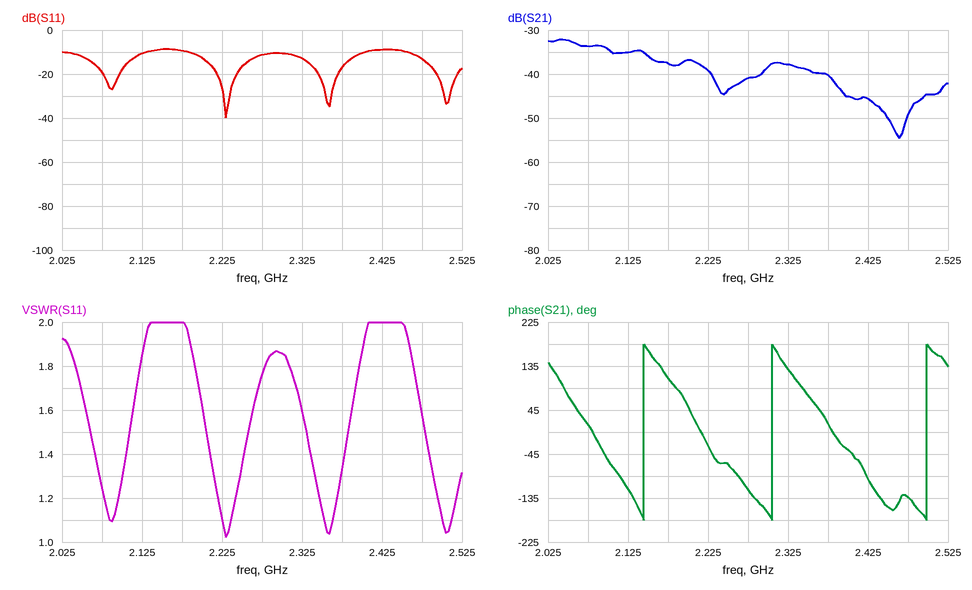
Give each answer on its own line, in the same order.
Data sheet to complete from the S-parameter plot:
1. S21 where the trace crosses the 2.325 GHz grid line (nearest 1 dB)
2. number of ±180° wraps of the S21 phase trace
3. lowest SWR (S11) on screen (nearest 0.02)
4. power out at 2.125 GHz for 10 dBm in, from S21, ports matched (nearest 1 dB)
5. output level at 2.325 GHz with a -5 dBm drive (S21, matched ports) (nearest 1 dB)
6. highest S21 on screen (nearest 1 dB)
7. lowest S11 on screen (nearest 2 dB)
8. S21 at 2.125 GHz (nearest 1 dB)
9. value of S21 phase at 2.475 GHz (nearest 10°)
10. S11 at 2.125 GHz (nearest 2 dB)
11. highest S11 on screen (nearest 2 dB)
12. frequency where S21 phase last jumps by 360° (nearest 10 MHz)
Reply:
-38 dB
3
1.02
-25 dBm
-43 dBm
-32 dB
-40 dB
-35 dB
-130°
-10 dB
-8 dB
2.50 GHz
